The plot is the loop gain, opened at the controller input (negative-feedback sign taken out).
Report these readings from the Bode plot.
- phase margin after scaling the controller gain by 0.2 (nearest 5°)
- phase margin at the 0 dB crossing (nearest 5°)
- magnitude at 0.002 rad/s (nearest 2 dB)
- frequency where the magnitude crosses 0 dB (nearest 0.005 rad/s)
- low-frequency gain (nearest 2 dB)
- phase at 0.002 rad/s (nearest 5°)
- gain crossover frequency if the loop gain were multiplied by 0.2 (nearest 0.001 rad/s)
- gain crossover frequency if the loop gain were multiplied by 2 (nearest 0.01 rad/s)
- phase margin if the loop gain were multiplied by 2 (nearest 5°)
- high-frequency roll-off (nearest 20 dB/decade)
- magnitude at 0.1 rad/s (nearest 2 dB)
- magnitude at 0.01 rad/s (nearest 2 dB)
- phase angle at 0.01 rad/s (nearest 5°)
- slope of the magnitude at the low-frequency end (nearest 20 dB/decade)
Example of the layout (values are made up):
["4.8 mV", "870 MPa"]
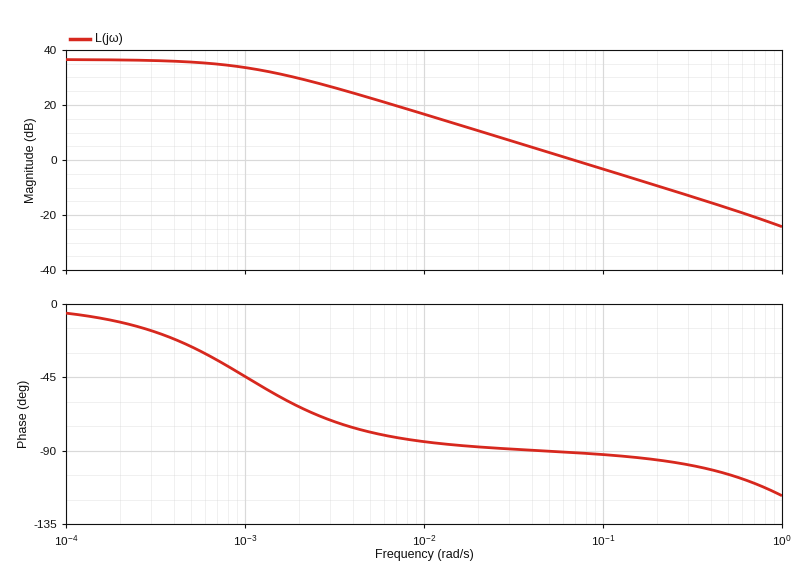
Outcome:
["95°", "90°", "30 dB", "0.070 rad/s", "36 dB", "-65°", "0.014 rad/s", "0.14 rad/s", "85°", "-20 dB/decade", "-4 dB", "16 dB", "-85°", "0 dB/decade"]
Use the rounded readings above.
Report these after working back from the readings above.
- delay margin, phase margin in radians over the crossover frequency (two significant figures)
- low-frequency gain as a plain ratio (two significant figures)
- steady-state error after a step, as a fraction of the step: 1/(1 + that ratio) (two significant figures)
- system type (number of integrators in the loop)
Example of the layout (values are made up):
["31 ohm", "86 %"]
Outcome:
["22 s", "63", "0.016", "0"]
